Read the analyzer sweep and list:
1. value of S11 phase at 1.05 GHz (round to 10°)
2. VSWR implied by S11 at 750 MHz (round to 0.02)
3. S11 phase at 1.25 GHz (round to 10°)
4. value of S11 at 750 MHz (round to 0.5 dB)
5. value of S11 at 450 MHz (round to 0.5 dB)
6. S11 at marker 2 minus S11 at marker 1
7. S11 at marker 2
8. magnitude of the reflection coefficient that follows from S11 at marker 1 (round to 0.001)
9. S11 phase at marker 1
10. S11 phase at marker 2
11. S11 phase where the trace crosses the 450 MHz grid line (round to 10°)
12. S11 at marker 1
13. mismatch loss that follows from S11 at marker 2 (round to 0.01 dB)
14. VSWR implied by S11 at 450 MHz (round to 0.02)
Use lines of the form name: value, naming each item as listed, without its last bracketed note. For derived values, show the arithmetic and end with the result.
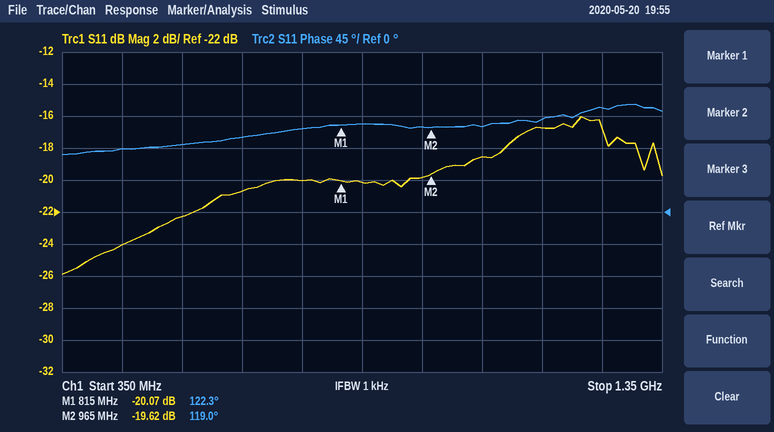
value of S11 phase at 1.05 GHz: 120°
VSWR implied by S11 at 750 MHz: |Γ| = 10^(-20/20) = 0.1000; VSWR = (1 + 0.1000)/(1 − 0.1000) ≈ 1.22
S11 phase at 1.25 GHz: 150°
value of S11 at 750 MHz: -20.0 dB
value of S11 at 450 MHz: -24.0 dB
S11 at marker 2 minus S11 at marker 1: -19.62 − (-20.07) = 0.45 dB
S11 at marker 2: -19.62 dB
magnitude of the reflection coefficient that follows from S11 at marker 1: 10^(-20.07/20) ≈ 0.099
S11 phase at marker 1: 122.3°
S11 phase at marker 2: 119.0°
S11 phase where the trace crosses the 450 MHz grid line: 90°
S11 at marker 1: -20.07 dB
mismatch loss that follows from S11 at marker 2: −10 log10(1 − 10^(-19.62/10)) ≈ 0.05 dB
VSWR implied by S11 at 450 MHz: |Γ| = 10^(-24/20) = 0.0631; VSWR = (1 + 0.0631)/(1 − 0.0631) ≈ 1.13, so 1.14 to the nearest 0.02
